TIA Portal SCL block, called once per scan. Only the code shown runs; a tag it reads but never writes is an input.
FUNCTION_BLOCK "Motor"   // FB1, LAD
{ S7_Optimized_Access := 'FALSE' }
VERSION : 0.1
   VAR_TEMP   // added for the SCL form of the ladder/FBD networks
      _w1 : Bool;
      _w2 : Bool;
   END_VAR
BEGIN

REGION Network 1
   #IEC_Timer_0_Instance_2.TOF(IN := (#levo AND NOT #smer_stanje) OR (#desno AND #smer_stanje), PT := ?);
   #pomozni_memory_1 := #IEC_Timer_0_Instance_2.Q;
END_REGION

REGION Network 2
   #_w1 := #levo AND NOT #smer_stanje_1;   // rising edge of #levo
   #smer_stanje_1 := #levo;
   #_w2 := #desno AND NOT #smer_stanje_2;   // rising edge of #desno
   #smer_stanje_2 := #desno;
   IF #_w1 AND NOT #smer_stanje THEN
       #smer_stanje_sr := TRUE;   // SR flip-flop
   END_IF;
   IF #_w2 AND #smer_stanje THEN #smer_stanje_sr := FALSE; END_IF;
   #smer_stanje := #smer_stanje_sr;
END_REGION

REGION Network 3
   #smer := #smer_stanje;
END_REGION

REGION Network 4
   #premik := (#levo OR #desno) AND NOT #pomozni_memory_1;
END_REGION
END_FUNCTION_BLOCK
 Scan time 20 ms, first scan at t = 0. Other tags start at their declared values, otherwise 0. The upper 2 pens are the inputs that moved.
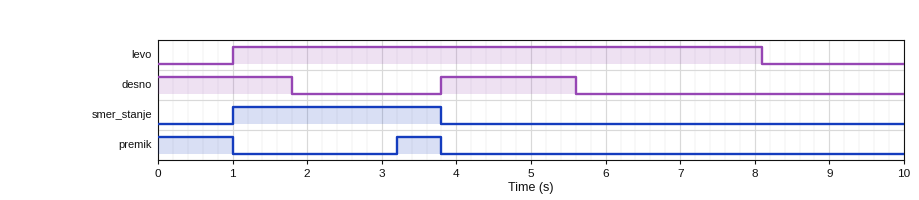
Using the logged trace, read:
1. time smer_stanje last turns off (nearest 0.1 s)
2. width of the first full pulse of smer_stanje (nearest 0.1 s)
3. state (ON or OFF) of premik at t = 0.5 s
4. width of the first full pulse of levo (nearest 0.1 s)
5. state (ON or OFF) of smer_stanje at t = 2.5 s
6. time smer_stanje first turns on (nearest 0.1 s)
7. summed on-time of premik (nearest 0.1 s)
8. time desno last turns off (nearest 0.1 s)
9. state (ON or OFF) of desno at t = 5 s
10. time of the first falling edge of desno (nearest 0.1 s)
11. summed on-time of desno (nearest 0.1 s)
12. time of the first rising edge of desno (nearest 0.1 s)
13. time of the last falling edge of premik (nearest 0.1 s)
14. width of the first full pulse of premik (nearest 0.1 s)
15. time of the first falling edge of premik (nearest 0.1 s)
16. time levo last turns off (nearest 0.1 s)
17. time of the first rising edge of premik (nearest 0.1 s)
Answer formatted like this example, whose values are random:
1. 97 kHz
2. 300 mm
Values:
1. 3.8 s
2. 2.8 s
3. ON
4. 7.1 s
5. ON
6. 1.0 s
7. 1.6 s
8. 5.6 s
9. ON
10. 1.8 s
11. 3.6 s
12. 3.8 s
13. 3.8 s
14. 0.6 s
15. 1.0 s
16. 8.1 s
17. 3.2 s
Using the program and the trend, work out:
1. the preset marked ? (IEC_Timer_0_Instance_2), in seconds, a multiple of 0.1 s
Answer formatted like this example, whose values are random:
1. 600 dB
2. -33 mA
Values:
1. 1.4 s
